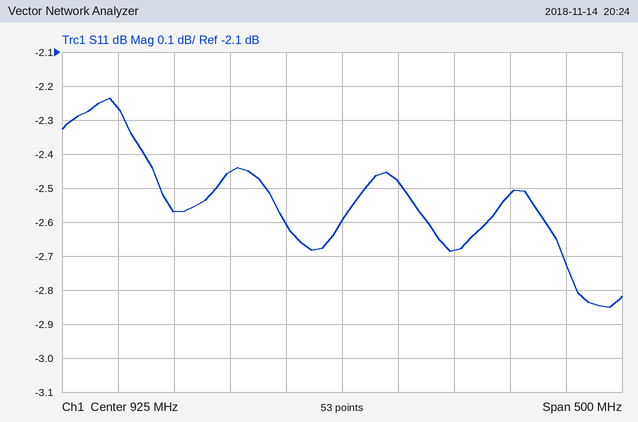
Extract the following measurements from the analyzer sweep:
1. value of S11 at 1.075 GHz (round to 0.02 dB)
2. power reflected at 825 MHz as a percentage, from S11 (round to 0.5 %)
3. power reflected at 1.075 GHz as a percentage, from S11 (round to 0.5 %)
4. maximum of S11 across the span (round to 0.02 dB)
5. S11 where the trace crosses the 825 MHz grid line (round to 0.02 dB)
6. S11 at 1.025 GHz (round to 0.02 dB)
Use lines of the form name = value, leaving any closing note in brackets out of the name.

value of S11 at 1.075 GHz = -2.52 dB
power reflected at 825 MHz as a percentage, from S11 = 57.0 %
power reflected at 1.075 GHz as a percentage, from S11 = 56.0 %
maximum of S11 across the span = -2.24 dB
S11 where the trace crosses the 825 MHz grid line = -2.46 dB
S11 at 1.025 GHz = -2.68 dB
